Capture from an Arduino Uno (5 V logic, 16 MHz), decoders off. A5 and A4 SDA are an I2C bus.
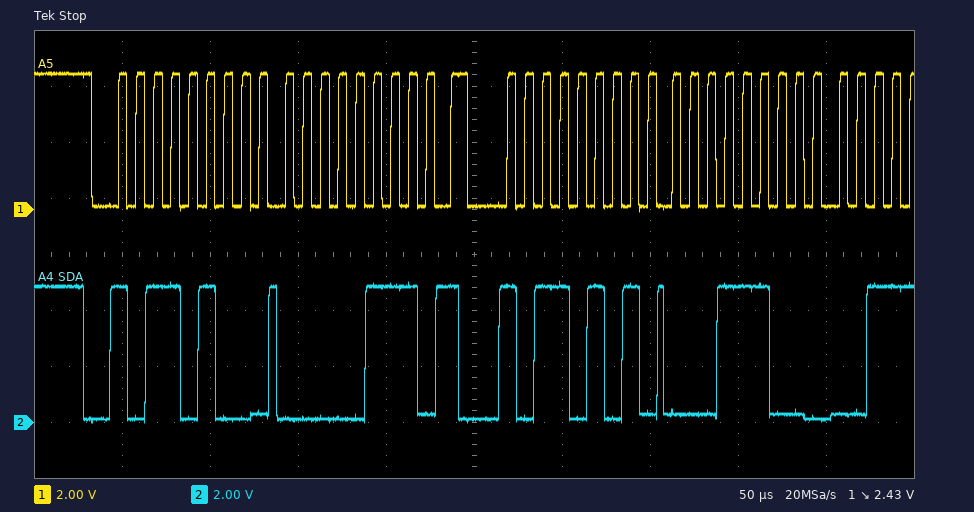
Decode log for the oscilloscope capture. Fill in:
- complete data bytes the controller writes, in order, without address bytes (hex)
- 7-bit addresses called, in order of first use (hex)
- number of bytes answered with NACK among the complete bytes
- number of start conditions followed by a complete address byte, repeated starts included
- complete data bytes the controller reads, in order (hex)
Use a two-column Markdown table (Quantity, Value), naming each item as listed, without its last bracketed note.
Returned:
| Quantity | Value |
|---|---|
| complete data bytes the controller writes, in order, without address bytes | 07 |
| 7-bit addresses called, in order of first use | 0x5A |
| number of bytes answered with NACK among the complete bytes | 0 |
| number of start conditions followed by a complete address byte, repeated starts included | 2 |
| complete data bytes the controller reads, in order | 1C |
